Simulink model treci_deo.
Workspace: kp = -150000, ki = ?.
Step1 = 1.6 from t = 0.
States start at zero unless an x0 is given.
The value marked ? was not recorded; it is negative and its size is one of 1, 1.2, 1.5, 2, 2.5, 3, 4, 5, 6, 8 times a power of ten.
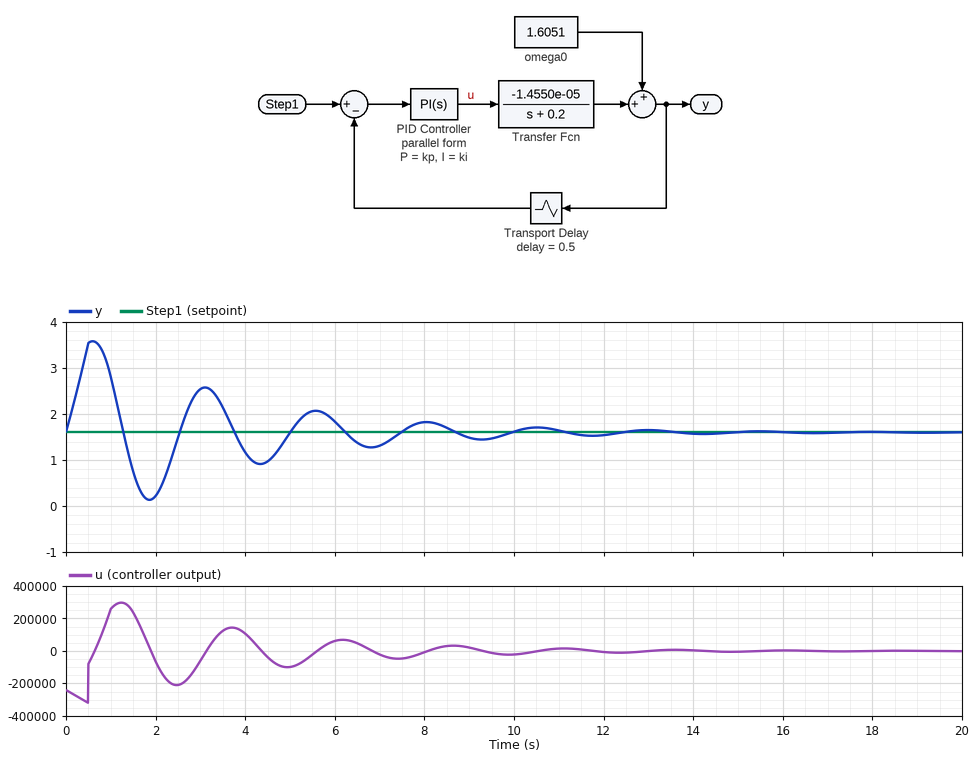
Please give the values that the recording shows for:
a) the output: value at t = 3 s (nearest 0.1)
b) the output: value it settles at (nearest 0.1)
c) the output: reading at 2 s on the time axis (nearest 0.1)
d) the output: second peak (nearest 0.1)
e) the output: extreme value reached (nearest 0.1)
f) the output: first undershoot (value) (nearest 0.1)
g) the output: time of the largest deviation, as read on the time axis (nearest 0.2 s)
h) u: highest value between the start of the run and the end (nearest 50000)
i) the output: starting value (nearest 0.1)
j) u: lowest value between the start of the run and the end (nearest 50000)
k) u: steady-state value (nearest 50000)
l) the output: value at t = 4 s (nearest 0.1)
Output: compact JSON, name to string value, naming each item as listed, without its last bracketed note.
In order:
{"the output: value at t = 3 s": "2.5", "the output: value it settles at": "1.6", "the output: reading at 2 s on the time axis": "0.2", "the output: second peak": "2.6", "the output: extreme value reached": "3.6", "the output: first undershoot (value)": "0.1", "the output: time of the largest deviation, as read on the time axis": "0.6 s", "u: highest value between the start of the run and the end": "300000", "the output: starting value": "1.6", "u: lowest value between the start of the run and the end": "-300000", "u: steady-state value": "0", "the output: value at t = 4 s": "1.2"}
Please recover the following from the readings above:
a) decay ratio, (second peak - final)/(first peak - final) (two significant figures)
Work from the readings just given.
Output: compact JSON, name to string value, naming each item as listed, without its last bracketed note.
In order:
{"decay ratio, (second peak - final)/(first peak - final)": "0.50"}
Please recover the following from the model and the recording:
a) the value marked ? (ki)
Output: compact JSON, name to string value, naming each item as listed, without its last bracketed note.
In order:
{"the value marked ?": "-100000"}
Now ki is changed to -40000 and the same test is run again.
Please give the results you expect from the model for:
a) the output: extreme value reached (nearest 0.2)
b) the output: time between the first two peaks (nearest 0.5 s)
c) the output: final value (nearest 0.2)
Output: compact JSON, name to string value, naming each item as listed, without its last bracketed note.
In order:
{"the output: extreme value reached": "3.4", "the output: time between the first two peaks": "2.5 s", "the output: final value": "1.6"}
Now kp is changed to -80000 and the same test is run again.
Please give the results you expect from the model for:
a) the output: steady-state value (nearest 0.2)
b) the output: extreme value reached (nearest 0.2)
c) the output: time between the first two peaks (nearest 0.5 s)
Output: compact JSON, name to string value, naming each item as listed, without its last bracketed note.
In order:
{"the output: steady-state value": "1.6", "the output: extreme value reached": "3.0", "the output: time between the first two peaks": "4.0 s"}
